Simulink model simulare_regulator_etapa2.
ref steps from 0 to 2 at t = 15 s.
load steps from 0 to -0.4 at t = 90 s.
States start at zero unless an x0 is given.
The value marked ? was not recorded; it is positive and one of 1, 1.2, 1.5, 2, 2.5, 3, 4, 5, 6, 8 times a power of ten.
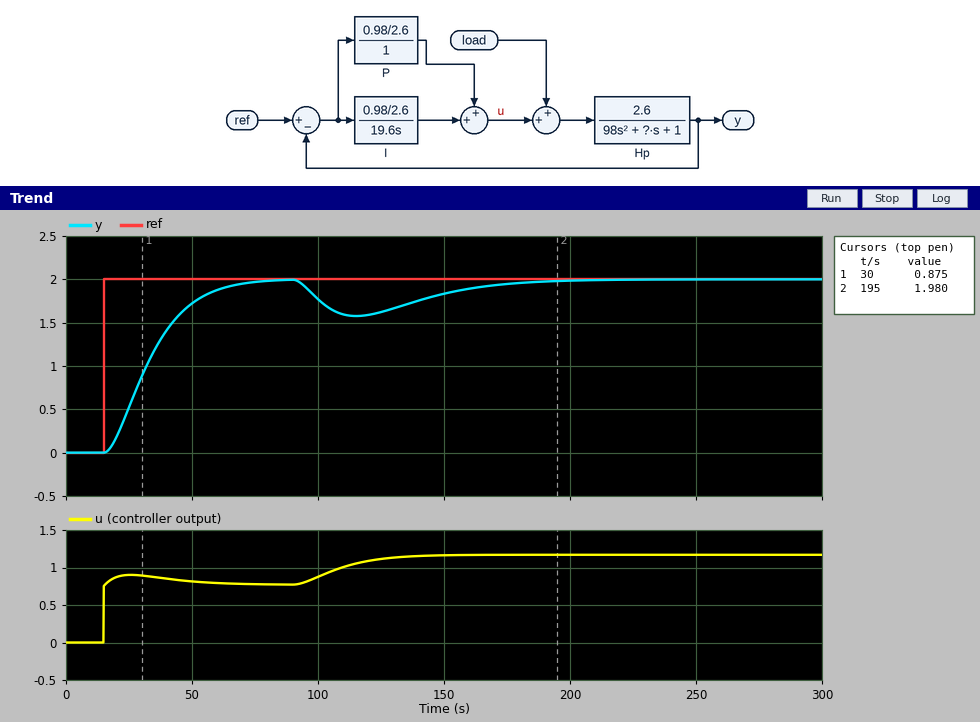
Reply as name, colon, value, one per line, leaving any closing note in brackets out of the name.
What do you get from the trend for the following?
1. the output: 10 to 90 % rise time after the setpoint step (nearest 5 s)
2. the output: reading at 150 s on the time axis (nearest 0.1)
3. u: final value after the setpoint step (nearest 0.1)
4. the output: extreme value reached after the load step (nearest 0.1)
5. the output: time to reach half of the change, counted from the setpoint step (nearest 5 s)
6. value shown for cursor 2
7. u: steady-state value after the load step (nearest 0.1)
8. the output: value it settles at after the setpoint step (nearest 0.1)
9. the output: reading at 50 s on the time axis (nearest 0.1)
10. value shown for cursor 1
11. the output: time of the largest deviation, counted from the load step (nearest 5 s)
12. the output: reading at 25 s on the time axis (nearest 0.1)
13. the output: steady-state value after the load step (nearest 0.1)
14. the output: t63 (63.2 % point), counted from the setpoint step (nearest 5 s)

the output: 10 to 90 % rise time after the setpoint step: 35 s
the output: reading at 150 s on the time axis: 1.8
u: final value after the setpoint step: 0.8
the output: extreme value reached after the load step: 1.6
the output: time to reach half of the change, counted from the setpoint step: 15 s
value shown for cursor 2: 1.980
u: steady-state value after the load step: 1.2
the output: value it settles at after the setpoint step: 2.0
the output: reading at 50 s on the time axis: 1.7
value shown for cursor 1: 0.875
the output: time of the largest deviation, counted from the load step: 25 s
the output: reading at 25 s on the time axis: 0.5
the output: steady-state value after the load step: 2.0
the output: t63 (63.2 % point), counted from the setpoint step: 20 s
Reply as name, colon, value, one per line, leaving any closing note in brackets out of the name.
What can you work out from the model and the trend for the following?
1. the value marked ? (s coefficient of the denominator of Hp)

the value marked ?: 25
